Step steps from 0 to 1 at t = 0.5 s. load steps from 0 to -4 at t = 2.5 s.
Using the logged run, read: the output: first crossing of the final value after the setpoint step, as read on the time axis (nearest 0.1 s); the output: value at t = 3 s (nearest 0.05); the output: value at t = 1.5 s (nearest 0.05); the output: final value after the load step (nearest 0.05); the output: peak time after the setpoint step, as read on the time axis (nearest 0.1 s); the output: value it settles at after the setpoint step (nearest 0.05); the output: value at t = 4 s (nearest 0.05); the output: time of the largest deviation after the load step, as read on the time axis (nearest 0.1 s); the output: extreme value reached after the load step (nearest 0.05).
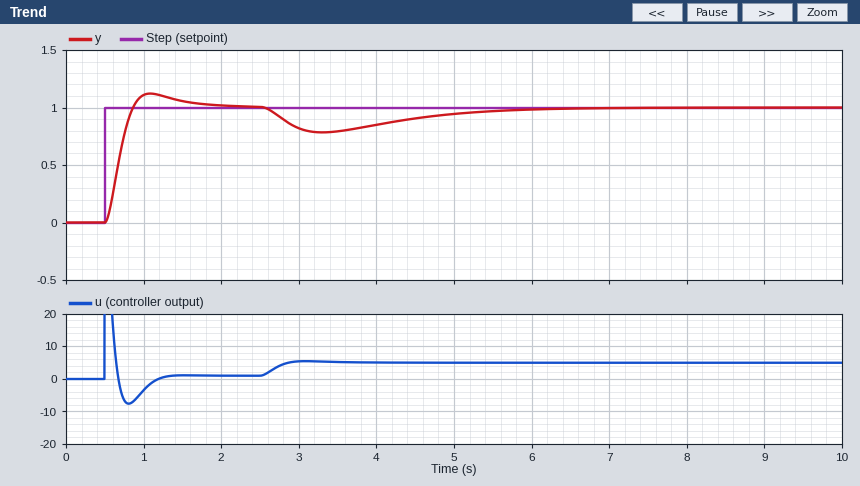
0.9 s
0.80
1.05
1.00
1.1 s
1.00
0.85
3.3 s
0.80
